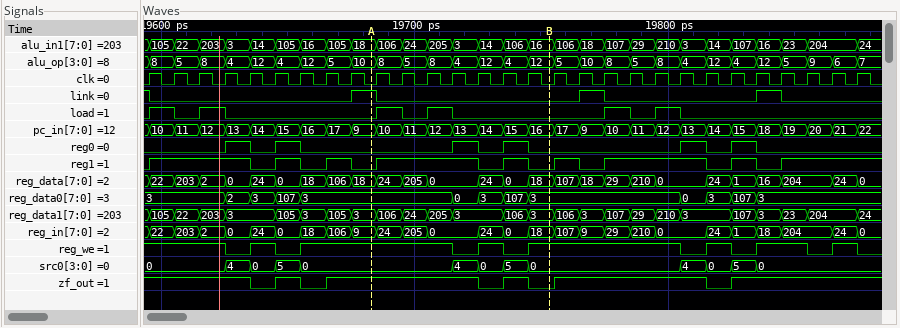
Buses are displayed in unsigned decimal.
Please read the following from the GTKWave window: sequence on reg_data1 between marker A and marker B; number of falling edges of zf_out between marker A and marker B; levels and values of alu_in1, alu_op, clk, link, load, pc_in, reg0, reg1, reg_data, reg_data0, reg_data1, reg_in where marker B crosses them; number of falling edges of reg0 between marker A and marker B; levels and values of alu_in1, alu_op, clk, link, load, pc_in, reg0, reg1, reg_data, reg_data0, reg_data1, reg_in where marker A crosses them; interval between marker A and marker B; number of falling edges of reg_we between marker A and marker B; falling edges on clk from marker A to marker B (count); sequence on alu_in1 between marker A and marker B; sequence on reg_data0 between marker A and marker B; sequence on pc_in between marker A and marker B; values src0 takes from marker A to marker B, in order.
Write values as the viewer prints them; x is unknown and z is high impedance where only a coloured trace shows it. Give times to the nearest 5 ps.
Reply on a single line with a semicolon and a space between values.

3, 106, 24, 205, 3, 106, 3; 2; alu_in1=16, alu_op=12, clk=0, link=0, load=0, pc_in=16, reg0=0, reg1=0, reg_data=18, reg_data0=3, reg_data1=3, reg_in=18; 2; alu_in1=18, alu_op=10, clk=0, link=1, load=0, pc_in=9, reg0=0, reg1=0, reg_data=18, reg_data0=3, reg_data1=3, reg_in=9; 70 ps; 2; 7; 18, 106, 24, 205, 3, 14, 106, 16; 3, 0, 3, 107, 3; 9, 10, 11, 12, 13, 14, 15, 16; 0, 4, 0, 5, 0
